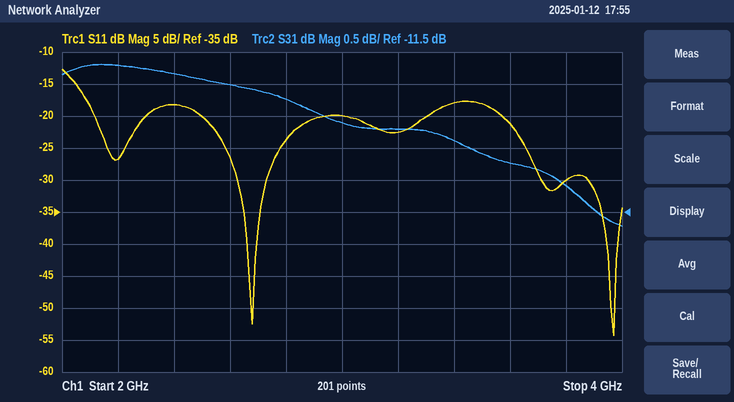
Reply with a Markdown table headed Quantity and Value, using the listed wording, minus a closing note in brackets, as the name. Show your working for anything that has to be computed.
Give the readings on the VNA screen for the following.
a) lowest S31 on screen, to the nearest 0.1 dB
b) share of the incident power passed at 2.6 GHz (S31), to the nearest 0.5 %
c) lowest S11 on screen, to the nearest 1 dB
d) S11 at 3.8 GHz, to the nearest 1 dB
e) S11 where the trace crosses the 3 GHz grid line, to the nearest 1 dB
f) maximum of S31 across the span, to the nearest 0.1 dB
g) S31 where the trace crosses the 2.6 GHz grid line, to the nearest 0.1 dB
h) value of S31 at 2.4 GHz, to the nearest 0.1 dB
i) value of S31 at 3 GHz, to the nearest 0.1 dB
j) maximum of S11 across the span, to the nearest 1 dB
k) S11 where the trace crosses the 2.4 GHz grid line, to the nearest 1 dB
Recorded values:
| Quantity | Value |
|---|---|
| lowest S31 on screen, to the nearest 0.1 dB | -11.7 dB |
| share of the incident power passed at 2.6 GHz (S31), to the nearest 0.5 % | 10^(-9.5/10) ≈ 11.2 %, so 11.0 % to the nearest 0.5 % |
| lowest S11 on screen, to the nearest 1 dB | -54 dB |
| S11 at 3.8 GHz, to the nearest 1 dB | -30 dB |
| S11 where the trace crosses the 3 GHz grid line, to the nearest 1 dB | -20 dB |
| maximum of S31 across the span, to the nearest 0.1 dB | -9.2 dB |
| S31 where the trace crosses the 2.6 GHz grid line, to the nearest 0.1 dB | -9.5 dB |
| value of S31 at 2.4 GHz, to the nearest 0.1 dB | -9.3 dB |
| value of S31 at 3 GHz, to the nearest 0.1 dB | -10.1 dB |
| maximum of S11 across the span, to the nearest 1 dB | -13 dB |
| S11 where the trace crosses the 2.4 GHz grid line, to the nearest 1 dB | -18 dB |
